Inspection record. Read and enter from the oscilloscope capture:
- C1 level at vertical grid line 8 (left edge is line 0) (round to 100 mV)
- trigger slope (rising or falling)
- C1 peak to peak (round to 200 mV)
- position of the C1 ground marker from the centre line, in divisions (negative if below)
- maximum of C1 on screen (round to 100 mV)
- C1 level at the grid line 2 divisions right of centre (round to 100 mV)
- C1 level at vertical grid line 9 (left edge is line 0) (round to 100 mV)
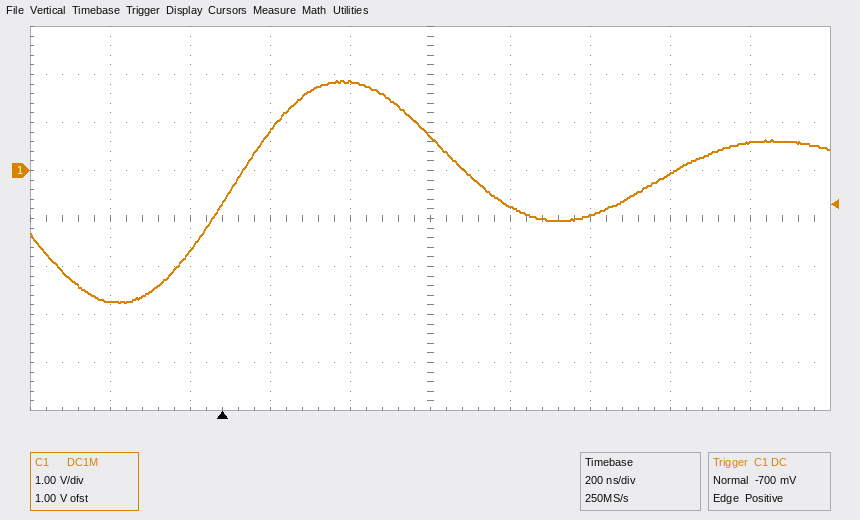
-100 mV
rising
4.6 V
+1.0 div
1.9 V
-900 mV
600 mV
